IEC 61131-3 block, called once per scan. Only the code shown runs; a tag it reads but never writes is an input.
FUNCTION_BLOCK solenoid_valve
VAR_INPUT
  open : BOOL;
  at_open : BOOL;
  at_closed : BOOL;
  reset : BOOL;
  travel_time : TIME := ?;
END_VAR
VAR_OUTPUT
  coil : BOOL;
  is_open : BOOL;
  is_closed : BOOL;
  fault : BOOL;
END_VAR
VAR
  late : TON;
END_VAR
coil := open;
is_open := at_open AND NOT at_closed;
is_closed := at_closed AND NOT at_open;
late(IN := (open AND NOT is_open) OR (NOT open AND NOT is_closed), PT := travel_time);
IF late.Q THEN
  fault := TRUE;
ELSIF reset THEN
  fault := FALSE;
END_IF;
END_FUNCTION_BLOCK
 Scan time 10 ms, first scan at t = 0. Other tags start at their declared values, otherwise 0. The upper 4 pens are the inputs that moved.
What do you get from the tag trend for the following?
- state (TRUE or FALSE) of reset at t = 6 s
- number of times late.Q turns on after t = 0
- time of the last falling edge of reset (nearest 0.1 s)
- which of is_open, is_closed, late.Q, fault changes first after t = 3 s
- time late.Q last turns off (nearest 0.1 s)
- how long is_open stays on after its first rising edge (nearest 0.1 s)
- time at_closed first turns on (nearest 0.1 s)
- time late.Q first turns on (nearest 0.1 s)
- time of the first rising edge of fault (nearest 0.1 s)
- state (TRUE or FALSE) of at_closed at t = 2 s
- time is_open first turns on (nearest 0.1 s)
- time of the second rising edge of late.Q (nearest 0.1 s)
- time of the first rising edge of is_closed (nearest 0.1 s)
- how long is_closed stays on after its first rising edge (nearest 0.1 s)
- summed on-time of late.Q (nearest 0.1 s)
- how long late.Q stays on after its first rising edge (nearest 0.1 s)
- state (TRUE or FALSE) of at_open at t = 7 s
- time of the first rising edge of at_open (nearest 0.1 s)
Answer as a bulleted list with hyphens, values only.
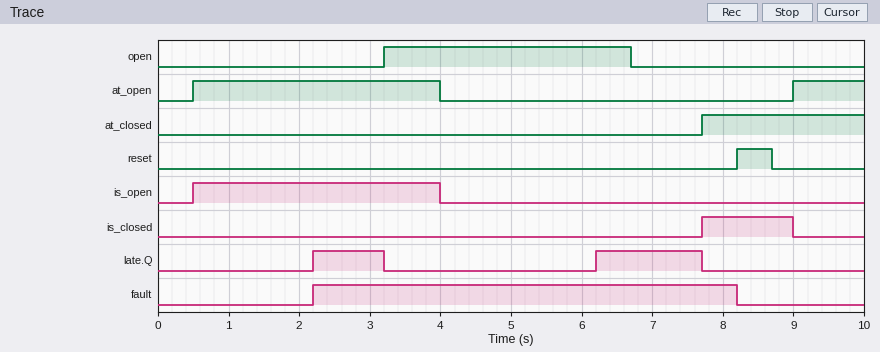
- FALSE
- 2
- 8.7 s
- late.Q
- 7.7 s
- 3.5 s
- 7.7 s
- 2.2 s
- 2.2 s
- FALSE
- 0.5 s
- 6.2 s
- 7.7 s
- 1.3 s
- 2.5 s
- 1.0 s
- FALSE
- 0.5 s
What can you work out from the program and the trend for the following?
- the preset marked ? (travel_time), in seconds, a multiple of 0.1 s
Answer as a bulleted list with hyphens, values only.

- 2.2 s
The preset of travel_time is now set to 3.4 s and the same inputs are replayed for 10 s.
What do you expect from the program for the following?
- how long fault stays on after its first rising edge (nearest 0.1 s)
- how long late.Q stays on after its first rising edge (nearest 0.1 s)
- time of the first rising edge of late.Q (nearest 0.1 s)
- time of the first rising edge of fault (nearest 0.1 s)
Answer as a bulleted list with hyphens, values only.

- 0.8 s
- 0.3 s
- 7.4 s
- 7.4 s
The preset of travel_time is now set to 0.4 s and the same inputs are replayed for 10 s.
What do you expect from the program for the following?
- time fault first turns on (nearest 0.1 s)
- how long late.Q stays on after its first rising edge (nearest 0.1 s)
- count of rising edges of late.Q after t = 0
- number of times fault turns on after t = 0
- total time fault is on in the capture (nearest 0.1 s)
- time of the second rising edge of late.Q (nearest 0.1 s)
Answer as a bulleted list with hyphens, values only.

- 0.4 s
- 2.8 s
- 3
- 2
- 8.4 s
- 4.4 s
